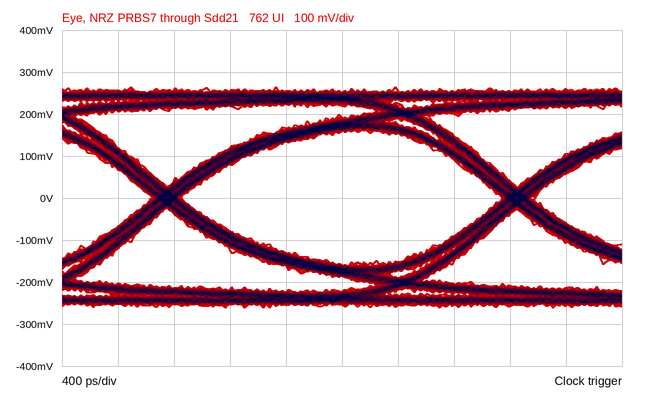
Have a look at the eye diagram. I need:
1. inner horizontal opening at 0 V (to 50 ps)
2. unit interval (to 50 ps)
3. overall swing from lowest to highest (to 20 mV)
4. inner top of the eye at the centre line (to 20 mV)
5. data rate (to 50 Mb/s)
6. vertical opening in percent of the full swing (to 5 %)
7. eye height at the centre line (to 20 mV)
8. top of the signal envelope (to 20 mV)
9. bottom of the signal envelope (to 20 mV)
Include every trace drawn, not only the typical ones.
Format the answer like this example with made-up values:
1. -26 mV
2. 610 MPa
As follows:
1. 2.30 ns
2. 2.50 ns
3. 520 mV
4. 160 mV
5. 400 Mb/s
6. 60 %
7. 320 mV
8. 260 mV
9. -260 mV
